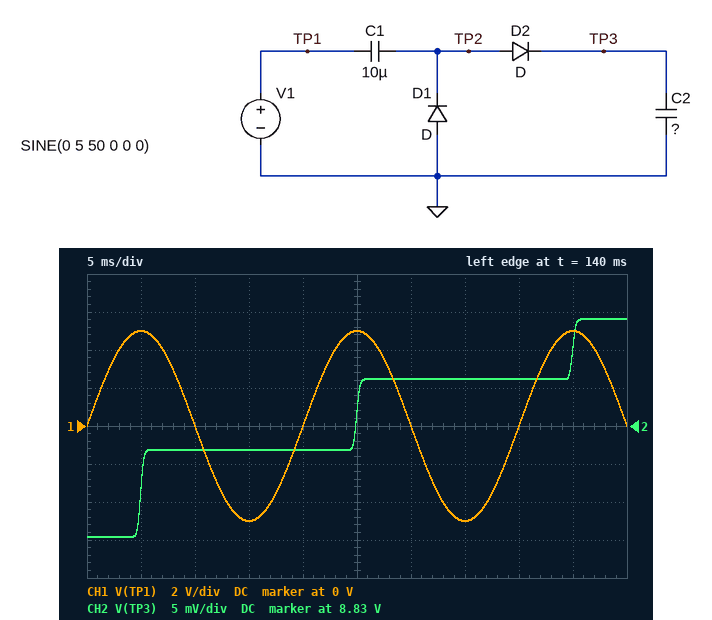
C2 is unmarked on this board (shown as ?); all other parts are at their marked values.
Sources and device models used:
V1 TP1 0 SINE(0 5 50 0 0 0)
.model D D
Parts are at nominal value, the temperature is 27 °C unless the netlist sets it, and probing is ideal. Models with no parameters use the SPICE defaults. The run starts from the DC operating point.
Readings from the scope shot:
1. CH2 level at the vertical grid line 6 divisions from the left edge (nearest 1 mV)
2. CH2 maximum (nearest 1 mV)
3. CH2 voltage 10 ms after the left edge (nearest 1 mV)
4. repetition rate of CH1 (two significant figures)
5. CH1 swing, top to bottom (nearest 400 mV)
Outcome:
8.836 V
8.844 V
8.827 V
50 Hz
10.0 V
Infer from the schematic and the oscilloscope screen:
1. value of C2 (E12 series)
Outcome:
2.2 µF
